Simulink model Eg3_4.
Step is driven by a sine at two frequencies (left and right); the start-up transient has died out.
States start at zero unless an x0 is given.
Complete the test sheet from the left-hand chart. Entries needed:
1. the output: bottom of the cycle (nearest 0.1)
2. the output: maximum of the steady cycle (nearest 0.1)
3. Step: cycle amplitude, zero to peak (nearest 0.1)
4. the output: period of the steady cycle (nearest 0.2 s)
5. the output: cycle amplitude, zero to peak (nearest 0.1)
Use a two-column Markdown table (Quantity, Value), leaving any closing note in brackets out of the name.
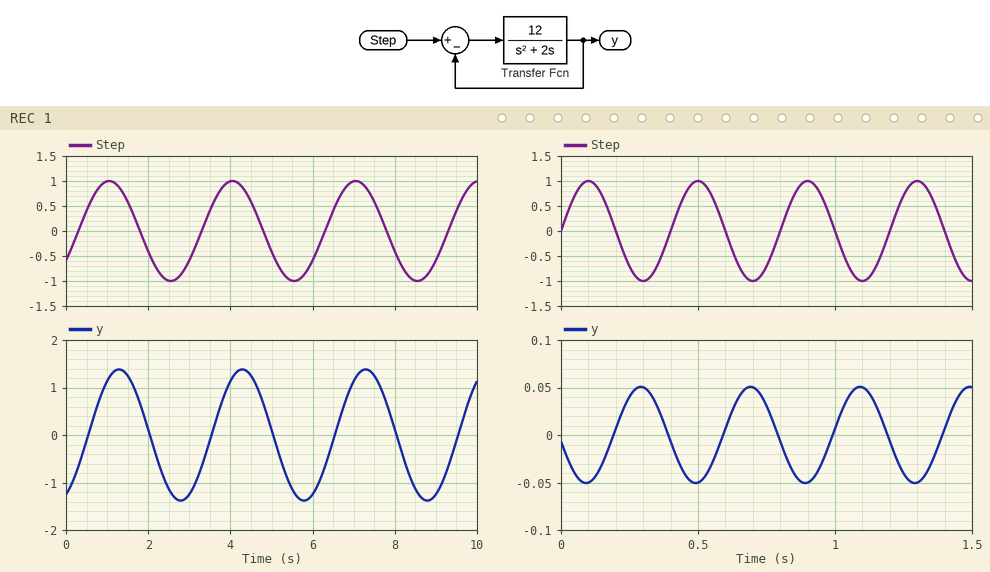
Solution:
| Quantity | Value |
|---|---|
| the output: bottom of the cycle | -1.4 |
| the output: maximum of the steady cycle | 1.4 |
| Step: cycle amplitude, zero to peak | 1.0 |
| the output: period of the steady cycle | 3.0 s |
| the output: cycle amplitude, zero to peak | 1.4 |
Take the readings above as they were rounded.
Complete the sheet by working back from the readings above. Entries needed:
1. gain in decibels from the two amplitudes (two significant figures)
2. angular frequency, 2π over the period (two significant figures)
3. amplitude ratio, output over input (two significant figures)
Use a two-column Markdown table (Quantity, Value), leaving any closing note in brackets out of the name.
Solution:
| Quantity | Value |
|---|---|
| gain in decibels from the two amplitudes | 2.9 dB |
| angular frequency, 2π over the period | 2.1 rad/s |
| amplitude ratio, output over input | 1.4 |
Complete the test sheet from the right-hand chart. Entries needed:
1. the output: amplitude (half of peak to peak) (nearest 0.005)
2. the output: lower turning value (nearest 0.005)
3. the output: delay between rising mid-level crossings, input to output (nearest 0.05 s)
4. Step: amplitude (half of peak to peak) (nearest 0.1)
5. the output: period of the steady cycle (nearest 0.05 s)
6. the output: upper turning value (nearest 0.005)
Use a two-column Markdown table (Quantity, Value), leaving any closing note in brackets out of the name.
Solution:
| Quantity | Value |
|---|---|
| the output: amplitude (half of peak to peak) | 0.050 |
| the output: lower turning value | -0.050 |
| the output: delay between rising mid-level crossings, input to output | 0.20 s |
| Step: amplitude (half of peak to peak) | 1.0 |
| the output: period of the steady cycle | 0.40 s |
| the output: upper turning value | 0.050 |
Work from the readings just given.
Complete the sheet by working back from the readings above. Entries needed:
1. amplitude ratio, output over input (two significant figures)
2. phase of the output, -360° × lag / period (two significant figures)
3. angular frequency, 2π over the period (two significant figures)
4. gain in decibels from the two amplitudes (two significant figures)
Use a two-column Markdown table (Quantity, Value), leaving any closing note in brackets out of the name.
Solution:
| Quantity | Value |
|---|---|
| amplitude ratio, output over input | 0.050 |
| phase of the output, -360° × lag / period | -180° |
| angular frequency, 2π over the period | 16 rad/s |
| gain in decibels from the two amplitudes | -26 dB |
